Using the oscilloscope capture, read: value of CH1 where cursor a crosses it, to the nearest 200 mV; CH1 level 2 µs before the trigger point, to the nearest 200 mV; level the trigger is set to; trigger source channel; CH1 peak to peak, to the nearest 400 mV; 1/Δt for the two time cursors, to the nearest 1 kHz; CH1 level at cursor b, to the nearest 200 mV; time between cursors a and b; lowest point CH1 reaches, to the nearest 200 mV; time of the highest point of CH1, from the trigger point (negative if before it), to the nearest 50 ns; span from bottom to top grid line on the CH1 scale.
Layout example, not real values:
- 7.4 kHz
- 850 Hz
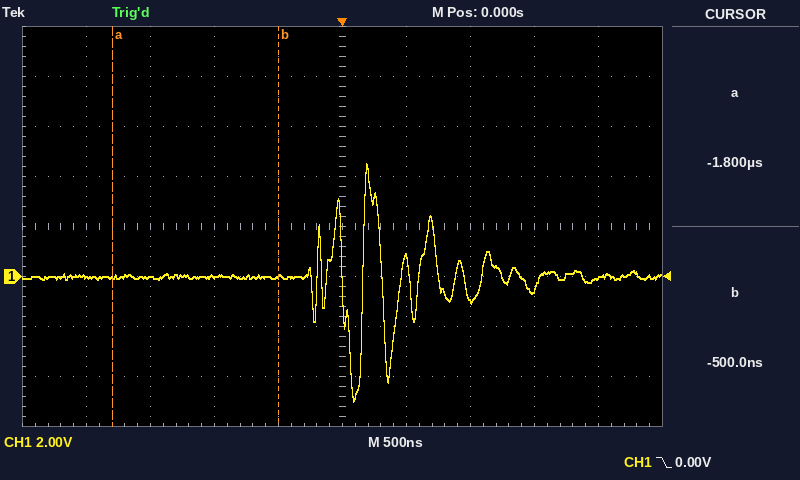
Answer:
- 0.0 V
- 0.0 V
- 0.00 V
- CH1
- 9.6 V
- 769 kHz
- 0.0 V
- 1.30 µs
- -5.0 V
- +200 ns
- 16 V
